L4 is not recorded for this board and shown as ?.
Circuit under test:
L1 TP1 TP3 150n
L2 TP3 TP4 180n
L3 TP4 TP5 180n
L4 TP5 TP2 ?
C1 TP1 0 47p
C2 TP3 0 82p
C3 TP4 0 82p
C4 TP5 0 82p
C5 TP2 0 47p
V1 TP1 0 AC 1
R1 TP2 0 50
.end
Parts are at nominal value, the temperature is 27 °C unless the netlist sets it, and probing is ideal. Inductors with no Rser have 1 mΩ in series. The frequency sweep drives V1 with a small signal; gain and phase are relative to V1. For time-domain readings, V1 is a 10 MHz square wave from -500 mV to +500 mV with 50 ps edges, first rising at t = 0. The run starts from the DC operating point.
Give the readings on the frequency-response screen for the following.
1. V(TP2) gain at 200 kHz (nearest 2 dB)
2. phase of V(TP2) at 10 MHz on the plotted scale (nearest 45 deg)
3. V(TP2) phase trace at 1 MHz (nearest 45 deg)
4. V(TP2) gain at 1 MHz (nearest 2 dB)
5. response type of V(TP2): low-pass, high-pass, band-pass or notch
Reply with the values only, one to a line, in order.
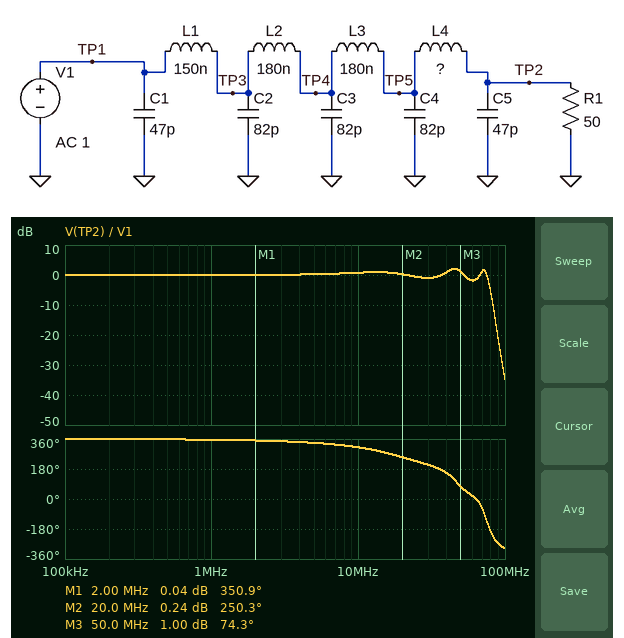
0 dB
315 deg
360 deg
0 dB
low-pass
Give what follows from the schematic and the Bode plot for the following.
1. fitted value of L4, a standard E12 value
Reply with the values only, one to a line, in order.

120 nH
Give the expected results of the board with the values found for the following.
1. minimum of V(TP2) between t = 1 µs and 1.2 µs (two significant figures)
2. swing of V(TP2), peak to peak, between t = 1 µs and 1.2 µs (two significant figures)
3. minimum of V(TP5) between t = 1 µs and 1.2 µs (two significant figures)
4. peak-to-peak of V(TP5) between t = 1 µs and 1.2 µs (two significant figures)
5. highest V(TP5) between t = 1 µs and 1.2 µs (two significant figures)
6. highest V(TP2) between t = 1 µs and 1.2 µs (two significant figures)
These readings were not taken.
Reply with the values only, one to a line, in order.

-740 mV
1.5 V
-660 mV
1.3 V
660 mV
740 mV
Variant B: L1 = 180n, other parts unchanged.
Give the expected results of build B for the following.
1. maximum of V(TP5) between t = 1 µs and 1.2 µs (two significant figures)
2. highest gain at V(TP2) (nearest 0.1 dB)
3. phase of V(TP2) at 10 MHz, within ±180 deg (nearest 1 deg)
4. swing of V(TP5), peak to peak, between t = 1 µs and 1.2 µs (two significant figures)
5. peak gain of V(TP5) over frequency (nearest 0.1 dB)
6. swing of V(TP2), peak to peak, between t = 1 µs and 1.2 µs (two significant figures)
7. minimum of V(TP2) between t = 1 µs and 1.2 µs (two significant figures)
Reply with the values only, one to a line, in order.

620 mV
1.3 dB
-52 deg
1.2 V
0.7 dB
1.4 V
-690 mV
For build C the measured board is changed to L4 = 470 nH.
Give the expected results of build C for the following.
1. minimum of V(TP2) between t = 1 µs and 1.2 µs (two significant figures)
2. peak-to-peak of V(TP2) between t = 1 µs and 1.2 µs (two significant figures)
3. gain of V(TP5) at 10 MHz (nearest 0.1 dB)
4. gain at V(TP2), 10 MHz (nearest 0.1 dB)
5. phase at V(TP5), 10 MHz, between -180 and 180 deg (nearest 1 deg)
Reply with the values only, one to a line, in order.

-620 mV
1.2 V
-0.4 dB
-1.2 dB
-29 deg
